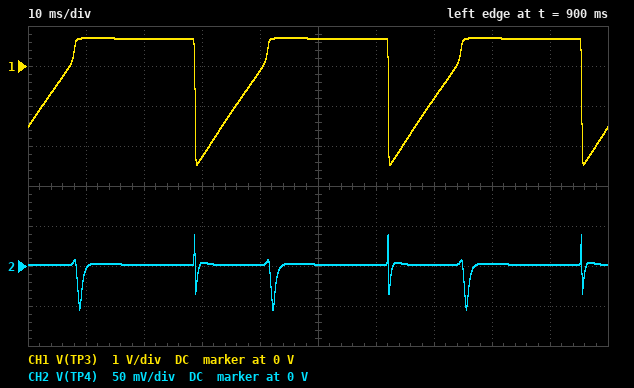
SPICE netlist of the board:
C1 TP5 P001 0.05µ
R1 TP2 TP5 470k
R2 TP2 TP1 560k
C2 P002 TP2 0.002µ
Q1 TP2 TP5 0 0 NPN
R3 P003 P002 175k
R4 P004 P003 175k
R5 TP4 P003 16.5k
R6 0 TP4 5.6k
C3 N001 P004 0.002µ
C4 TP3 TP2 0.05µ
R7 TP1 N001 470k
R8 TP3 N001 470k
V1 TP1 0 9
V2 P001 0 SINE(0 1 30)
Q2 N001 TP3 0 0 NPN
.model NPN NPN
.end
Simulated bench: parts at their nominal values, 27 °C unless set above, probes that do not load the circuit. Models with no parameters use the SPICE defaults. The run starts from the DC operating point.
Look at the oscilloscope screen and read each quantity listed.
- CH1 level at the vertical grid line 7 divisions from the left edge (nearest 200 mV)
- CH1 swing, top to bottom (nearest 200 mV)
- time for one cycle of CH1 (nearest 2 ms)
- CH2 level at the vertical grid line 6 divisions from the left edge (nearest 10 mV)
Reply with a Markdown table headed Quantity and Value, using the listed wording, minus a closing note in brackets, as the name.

| Quantity | Value |
|---|---|
| CH1 level at the vertical grid line 7 divisions from the left edge | -800 mV |
| CH1 swing, top to bottom | 3.2 V |
| time for one cycle of CH1 | 34 ms |
| CH2 level at the vertical grid line 6 divisions from the left edge | 0 V |
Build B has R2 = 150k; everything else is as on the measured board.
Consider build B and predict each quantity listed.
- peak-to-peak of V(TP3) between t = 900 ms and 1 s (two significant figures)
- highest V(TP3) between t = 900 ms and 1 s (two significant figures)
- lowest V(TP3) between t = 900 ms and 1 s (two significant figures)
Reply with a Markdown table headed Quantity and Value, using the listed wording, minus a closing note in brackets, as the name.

| Quantity | Value |
|---|---|
| peak-to-peak of V(TP3) between t = 900 ms and 1 s | 4.3 V |
| highest V(TP3) between t = 900 ms and 1 s | 710 mV |
| lowest V(TP3) between t = 900 ms and 1 s | -3.6 V |
